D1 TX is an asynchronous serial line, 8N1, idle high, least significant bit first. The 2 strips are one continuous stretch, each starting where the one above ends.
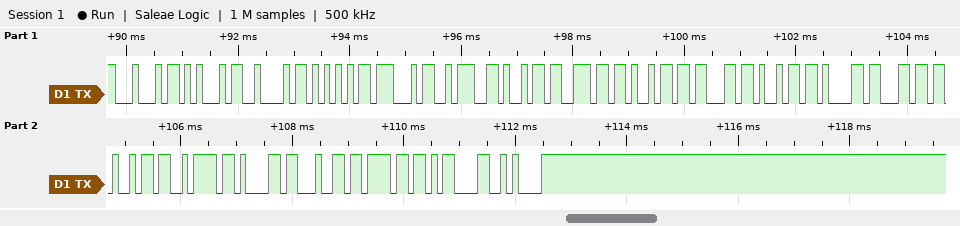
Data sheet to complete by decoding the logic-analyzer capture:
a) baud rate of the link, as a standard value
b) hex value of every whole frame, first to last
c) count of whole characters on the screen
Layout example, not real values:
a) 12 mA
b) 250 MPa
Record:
a) 9600 baud
b) 0x44 0x45 0x42 0x55 0x47 0x3A 0x69 0x6E 0x69 0x63 0x69 0x61 0x6C 0x69 0x7A 0x61 0x64 0x6F 0x0D 0x0A
c) 20
